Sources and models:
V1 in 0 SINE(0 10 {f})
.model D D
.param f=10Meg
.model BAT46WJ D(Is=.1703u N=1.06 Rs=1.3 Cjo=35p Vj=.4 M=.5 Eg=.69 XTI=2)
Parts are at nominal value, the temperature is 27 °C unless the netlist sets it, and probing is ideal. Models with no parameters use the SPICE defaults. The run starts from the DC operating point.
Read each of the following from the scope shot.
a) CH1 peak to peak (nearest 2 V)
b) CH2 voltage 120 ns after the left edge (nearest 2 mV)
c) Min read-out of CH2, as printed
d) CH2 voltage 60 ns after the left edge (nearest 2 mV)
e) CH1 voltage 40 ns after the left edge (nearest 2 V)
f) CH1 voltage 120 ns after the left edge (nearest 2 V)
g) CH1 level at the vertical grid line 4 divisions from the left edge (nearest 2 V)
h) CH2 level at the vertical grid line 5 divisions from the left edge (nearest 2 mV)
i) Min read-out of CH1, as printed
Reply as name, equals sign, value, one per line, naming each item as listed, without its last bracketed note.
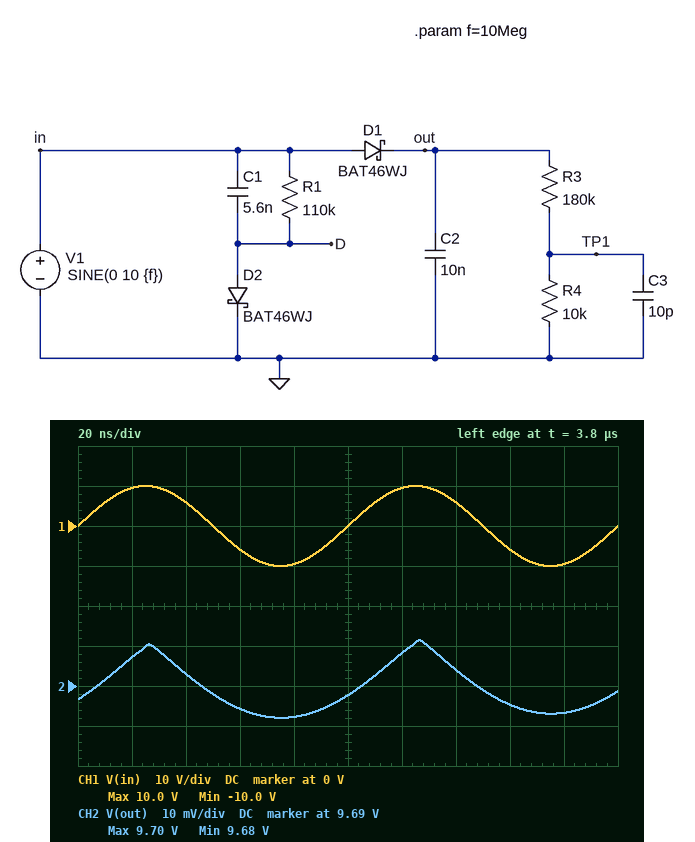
CH1 peak to peak = 20 V
CH2 voltage 120 ns after the left edge = 9.698 V
Min read-out of CH2, as printed = 9.68 V
CH2 voltage 60 ns after the left edge = 9.684 V
CH1 voltage 40 ns after the left edge = 6 V
CH1 voltage 120 ns after the left edge = 10 V
CH1 level at the vertical grid line 4 divisions from the left edge = -10 V
CH2 level at the vertical grid line 5 divisions from the left edge = 9.688 V
Min read-out of CH1, as printed = -10.0 V
